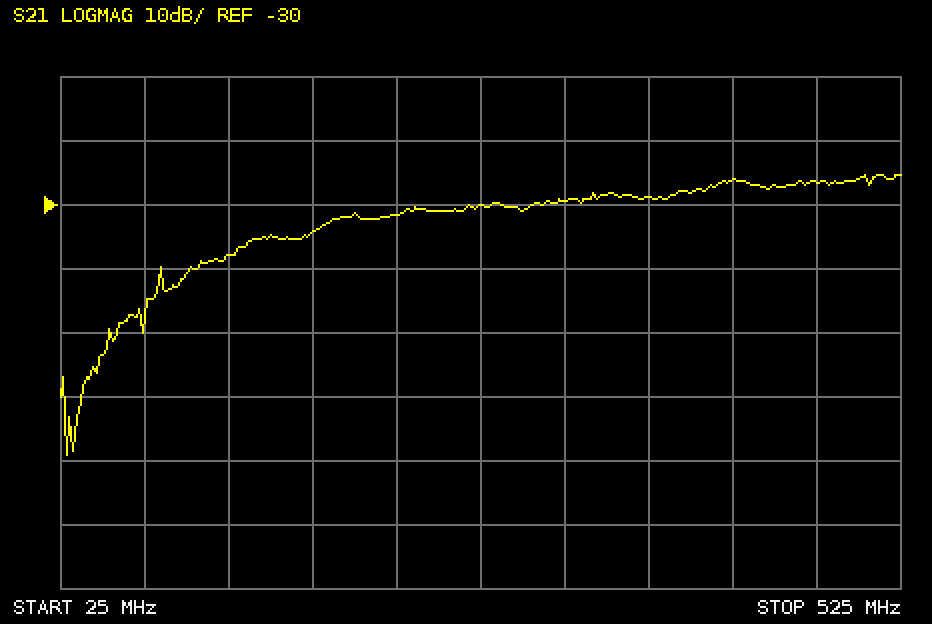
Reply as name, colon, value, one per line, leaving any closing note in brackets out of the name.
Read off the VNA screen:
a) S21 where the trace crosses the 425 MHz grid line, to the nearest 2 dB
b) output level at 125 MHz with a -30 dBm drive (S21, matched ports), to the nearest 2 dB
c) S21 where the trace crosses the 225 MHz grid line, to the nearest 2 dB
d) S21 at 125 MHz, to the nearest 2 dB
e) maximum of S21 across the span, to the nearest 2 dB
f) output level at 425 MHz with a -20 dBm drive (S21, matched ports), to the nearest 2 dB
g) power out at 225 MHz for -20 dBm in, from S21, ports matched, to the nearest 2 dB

S21 where the trace crosses the 425 MHz grid line, to the nearest 2 dB: -26 dB
output level at 125 MHz with a -30 dBm drive (S21, matched ports), to the nearest 2 dB: -68 dBm
S21 where the trace crosses the 225 MHz grid line, to the nearest 2 dB: -32 dB
S21 at 125 MHz, to the nearest 2 dB: -38 dB
maximum of S21 across the span, to the nearest 2 dB: -26 dB
output level at 425 MHz with a -20 dBm drive (S21, matched ports), to the nearest 2 dB: -46 dBm
power out at 225 MHz for -20 dBm in, from S21, ports matched, to the nearest 2 dB: -52 dBm
